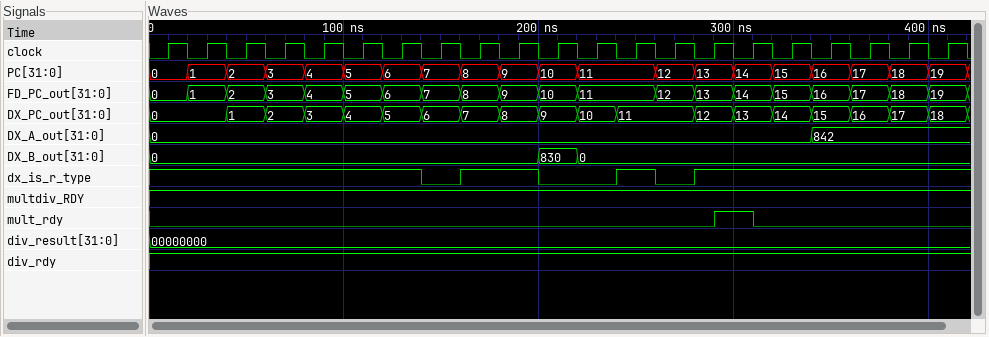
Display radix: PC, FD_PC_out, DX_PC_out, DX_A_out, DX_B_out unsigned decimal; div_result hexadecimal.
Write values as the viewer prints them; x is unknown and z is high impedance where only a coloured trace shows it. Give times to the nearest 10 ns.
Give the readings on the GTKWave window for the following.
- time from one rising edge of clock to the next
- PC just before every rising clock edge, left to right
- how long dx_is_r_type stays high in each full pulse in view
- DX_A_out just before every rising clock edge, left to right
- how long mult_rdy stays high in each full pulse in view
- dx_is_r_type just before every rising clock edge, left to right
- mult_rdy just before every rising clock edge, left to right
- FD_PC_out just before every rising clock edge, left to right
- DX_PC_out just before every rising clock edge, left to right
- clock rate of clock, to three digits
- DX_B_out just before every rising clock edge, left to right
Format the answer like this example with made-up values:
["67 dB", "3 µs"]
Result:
["20 ns", "0, 1, 2, 3, 4, 5, 6, 7, 8, 9, 10, 11, 11, 12, 13, 14, 15, 16, 17, 18, 19", "40 ns, 20 ns", "0, 0, 0, 0, 0, 0, 0, 0, 0, 0, 0, 0, 0, 0, 0, 0, 0, 842, 842, 842, 842", "20 ns", "1 1 1 1 1 1 1 0 1 1 0 0 1 0 1 1 1 1 1 1 1", "0 0 0 0 0 0 0 0 0 0 0 0 0 0 0 1 0 0 0 0 0", "0, 1, 2, 3, 4, 5, 6, 7, 8, 9, 10, 11, 11, 12, 13, 14, 15, 16, 17, 18, 19", "0, 0, 1, 2, 3, 4, 5, 6, 7, 8, 9, 10, 11, 11, 12, 13, 14, 15, 16, 17, 18", "50.0 MHz", "0, 0, 0, 0, 0, 0, 0, 0, 0, 0, 830, 0, 0, 0, 0, 0, 0, 0, 0, 0, 0"]
